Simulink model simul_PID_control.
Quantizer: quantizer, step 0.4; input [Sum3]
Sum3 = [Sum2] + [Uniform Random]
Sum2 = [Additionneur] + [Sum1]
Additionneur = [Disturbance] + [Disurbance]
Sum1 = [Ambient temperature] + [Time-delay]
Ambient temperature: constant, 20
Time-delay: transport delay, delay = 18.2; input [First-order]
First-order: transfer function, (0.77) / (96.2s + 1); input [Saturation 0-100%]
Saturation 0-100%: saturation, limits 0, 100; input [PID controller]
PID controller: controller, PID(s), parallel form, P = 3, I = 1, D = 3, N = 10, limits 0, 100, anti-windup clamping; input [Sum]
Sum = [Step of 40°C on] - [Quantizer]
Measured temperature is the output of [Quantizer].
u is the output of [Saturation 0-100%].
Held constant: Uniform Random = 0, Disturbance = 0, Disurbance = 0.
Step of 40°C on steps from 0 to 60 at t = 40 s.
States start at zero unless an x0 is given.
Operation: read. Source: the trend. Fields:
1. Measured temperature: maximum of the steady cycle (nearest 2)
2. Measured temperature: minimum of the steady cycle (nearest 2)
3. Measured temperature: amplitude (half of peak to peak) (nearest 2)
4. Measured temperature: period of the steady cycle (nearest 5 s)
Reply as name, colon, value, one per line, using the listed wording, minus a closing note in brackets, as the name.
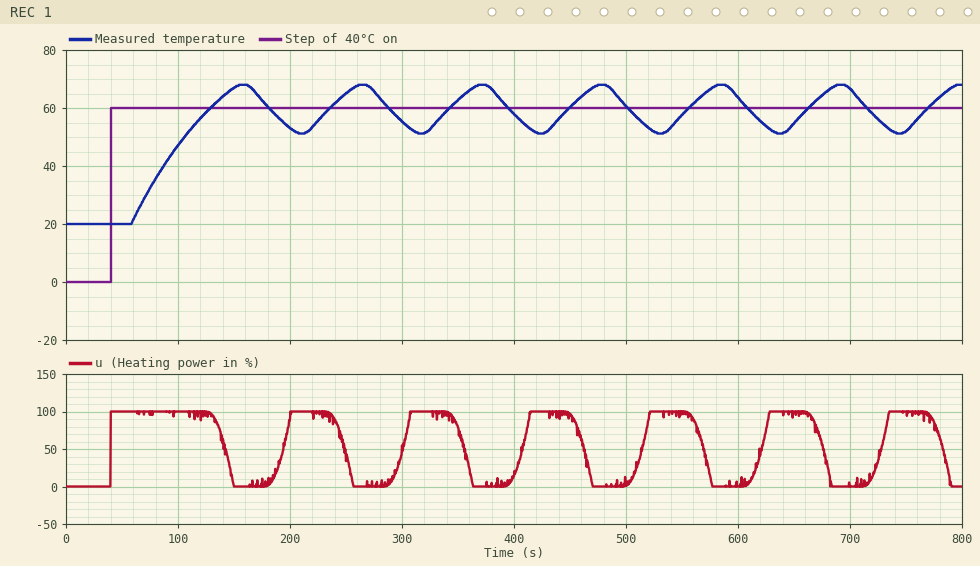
Measured temperature: maximum of the steady cycle: 68
Measured temperature: minimum of the steady cycle: 52
Measured temperature: amplitude (half of peak to peak): 8
Measured temperature: period of the steady cycle: 105 s
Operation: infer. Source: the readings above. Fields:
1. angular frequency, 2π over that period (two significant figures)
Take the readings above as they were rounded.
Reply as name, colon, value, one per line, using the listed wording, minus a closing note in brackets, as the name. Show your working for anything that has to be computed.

angular frequency, 2π over that period: 2π / 105 = 0.060 rad/s
